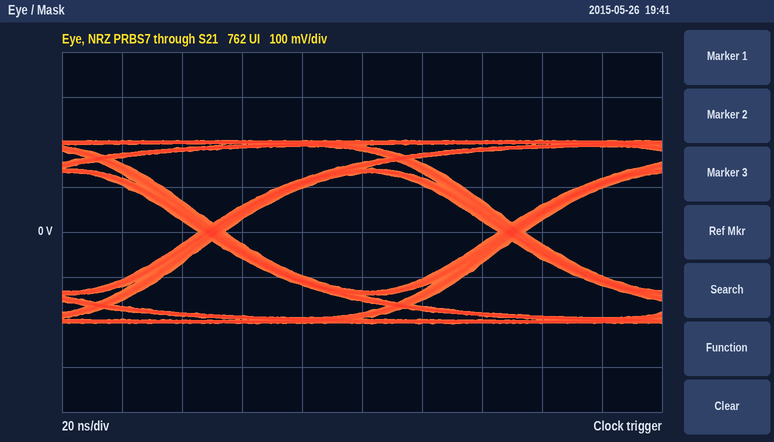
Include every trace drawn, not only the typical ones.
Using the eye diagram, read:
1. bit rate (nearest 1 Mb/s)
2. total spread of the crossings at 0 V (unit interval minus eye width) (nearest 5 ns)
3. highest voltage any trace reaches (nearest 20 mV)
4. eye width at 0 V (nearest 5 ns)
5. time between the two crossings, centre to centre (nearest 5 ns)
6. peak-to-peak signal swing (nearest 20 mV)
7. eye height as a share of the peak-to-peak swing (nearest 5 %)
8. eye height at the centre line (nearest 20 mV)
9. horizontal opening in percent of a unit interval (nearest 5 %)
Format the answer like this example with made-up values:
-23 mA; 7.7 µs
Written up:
10 Mb/s; 10 ns; 200 mV; 90 ns; 100 ns; 400 mV; 65 %; 260 mV; 90 %
